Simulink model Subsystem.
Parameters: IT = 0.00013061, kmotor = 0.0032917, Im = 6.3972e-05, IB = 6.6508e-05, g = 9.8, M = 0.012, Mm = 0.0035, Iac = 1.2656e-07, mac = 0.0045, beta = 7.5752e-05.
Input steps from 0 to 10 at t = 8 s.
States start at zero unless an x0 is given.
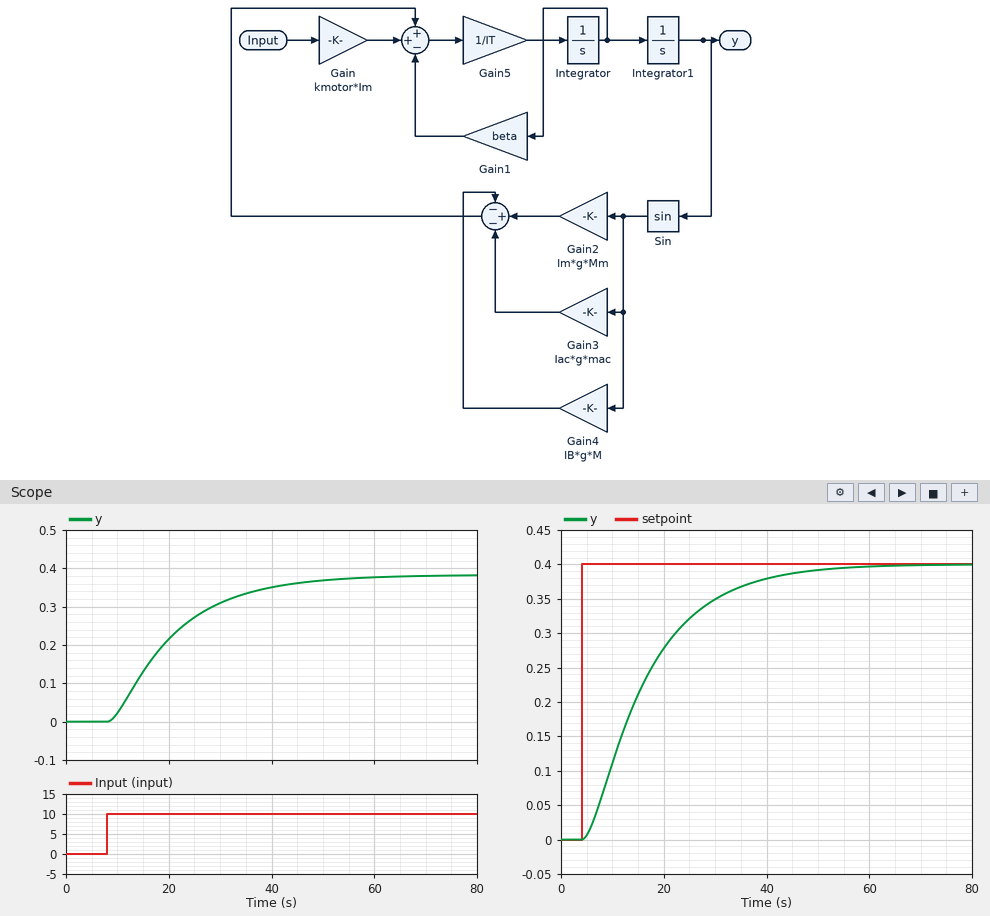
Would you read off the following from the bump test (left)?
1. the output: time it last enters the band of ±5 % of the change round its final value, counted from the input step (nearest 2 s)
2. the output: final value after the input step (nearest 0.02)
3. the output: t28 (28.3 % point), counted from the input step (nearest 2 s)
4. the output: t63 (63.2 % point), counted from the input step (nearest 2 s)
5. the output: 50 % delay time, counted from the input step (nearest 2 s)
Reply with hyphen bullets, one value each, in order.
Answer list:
- 38 s
- 0.38
- 6 s
- 14 s
- 10 s
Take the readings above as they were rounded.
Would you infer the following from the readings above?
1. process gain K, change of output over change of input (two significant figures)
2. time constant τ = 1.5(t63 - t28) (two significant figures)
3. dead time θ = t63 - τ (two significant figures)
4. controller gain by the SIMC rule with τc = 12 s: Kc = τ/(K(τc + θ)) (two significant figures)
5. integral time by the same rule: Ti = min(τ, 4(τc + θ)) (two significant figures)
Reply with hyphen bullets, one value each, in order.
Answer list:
- 0.038
- 12 s
- 2.0 s
- 23
- 12 s
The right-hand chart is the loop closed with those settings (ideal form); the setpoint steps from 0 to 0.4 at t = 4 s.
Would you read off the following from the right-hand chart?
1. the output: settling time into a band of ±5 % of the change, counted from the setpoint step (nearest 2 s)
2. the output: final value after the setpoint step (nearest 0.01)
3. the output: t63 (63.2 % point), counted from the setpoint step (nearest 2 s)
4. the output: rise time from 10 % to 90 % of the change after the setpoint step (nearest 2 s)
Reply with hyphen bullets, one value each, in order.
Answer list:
- 36 s
- 0.40
- 14 s
- 26 s
